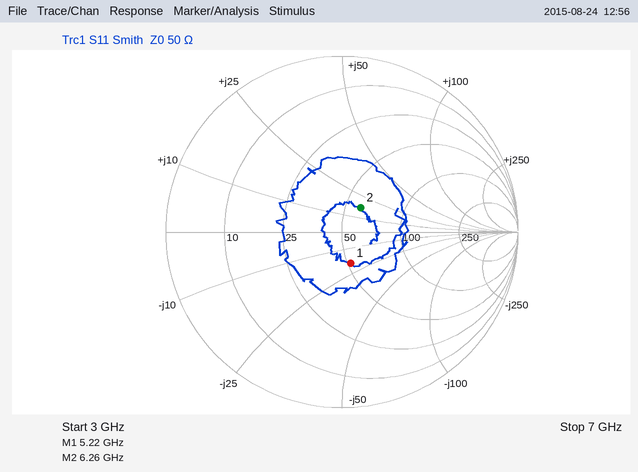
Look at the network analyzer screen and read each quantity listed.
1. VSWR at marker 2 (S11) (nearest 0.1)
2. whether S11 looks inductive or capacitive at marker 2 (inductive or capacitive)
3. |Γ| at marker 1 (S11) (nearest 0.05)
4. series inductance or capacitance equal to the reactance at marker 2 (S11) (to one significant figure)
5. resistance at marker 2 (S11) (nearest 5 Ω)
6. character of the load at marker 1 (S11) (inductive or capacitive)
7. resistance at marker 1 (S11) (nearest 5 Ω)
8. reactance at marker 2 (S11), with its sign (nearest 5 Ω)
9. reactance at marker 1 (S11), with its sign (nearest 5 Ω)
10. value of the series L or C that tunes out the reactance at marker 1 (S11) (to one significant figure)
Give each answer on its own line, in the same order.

1.4
inductive
0.20
400 pH
60 Ω
capacitive
50 Ω
+15 Ω
-20 Ω
600 pH
